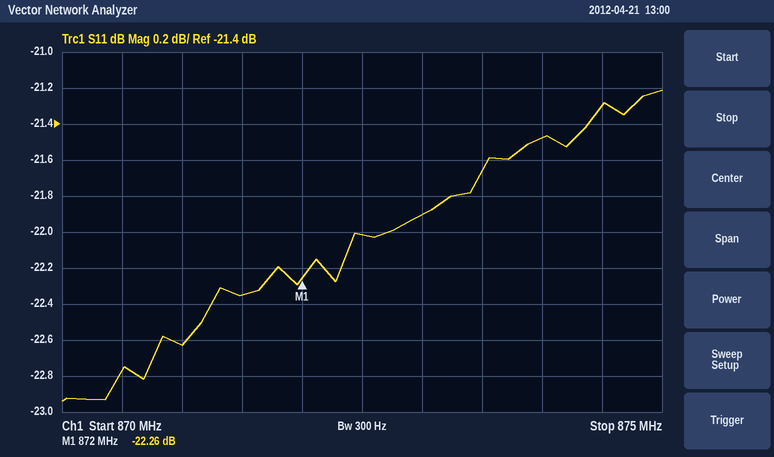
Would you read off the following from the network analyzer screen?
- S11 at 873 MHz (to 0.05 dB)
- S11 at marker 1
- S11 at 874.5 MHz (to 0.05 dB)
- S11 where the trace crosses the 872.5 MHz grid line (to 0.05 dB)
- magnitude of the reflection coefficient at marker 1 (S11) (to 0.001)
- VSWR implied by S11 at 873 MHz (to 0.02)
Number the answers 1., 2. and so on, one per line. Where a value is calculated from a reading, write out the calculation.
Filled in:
1. -21.90 dB
2. -22.26 dB
3. -21.30 dB
4. -22.00 dB
5. 10^(-22.26/20) ≈ 0.077
6. |Γ| = 10^(-21.9/20) = 0.0804; VSWR = (1 + 0.0804)/(1 − 0.0804) ≈ 1.17, so 1.18 to the nearest 0.02
